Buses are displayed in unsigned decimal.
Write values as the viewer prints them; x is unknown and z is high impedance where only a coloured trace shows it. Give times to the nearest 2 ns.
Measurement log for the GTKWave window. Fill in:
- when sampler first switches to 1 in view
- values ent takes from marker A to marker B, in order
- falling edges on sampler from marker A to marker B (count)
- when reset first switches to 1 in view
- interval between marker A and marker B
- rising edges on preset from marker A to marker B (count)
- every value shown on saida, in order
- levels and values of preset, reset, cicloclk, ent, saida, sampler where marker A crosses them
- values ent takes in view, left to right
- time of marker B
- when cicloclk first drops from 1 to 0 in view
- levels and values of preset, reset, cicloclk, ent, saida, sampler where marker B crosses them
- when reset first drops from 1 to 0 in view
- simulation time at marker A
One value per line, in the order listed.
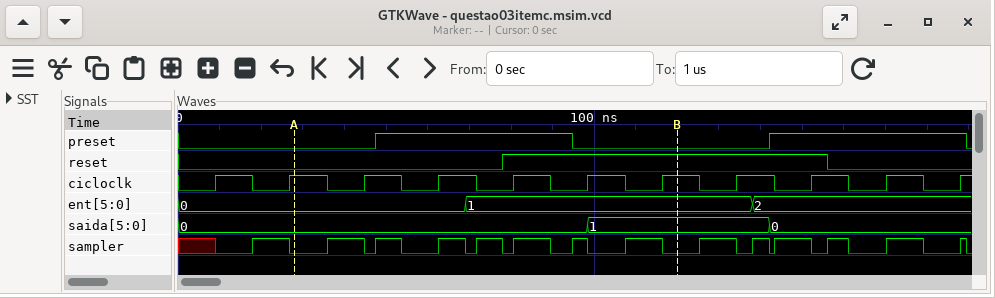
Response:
18 ns
0, 1
7
78 ns
92 ns
1
0, 1, 0
preset=0, reset=0, cicloclk=1, ent=0, saida=0, sampler=0
0, 1, 2
120 ns
18 ns
preset=0, reset=1, cicloclk=1, ent=1, saida=1, sampler=0
156 ns
28 ns
